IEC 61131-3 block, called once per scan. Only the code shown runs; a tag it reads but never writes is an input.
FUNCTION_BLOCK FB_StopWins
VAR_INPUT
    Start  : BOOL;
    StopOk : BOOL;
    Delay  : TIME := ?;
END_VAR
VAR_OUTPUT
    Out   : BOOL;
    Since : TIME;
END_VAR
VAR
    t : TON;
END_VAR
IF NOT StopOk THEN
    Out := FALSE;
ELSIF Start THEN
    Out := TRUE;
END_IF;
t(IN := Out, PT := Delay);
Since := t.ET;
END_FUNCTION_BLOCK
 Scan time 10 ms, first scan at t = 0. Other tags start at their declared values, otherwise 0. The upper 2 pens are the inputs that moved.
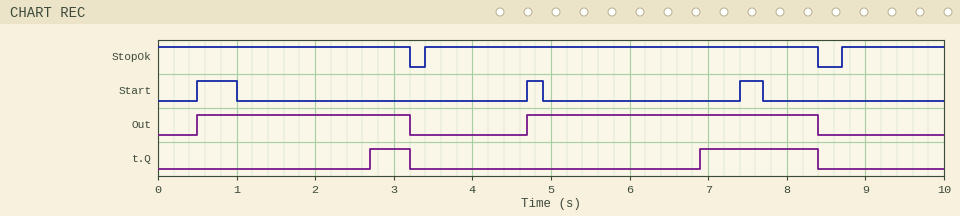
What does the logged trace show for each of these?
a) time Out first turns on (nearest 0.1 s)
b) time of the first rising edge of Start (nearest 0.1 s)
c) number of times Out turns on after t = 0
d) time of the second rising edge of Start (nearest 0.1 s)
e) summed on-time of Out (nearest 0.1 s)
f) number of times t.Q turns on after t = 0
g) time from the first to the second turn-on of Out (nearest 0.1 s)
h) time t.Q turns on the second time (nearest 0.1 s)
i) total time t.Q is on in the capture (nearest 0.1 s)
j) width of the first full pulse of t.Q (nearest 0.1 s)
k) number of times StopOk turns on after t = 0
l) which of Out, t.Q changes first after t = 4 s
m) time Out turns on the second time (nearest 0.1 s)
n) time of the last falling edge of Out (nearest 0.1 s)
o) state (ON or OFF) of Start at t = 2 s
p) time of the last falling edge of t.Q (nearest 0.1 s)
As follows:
0.5 s
0.5 s
2
4.7 s
6.4 s
2
4.2 s
6.9 s
2.0 s
0.5 s
2
Out
4.7 s
8.4 s
OFF
8.4 s
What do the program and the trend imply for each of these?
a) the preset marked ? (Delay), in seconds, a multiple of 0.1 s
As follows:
2.2 s
